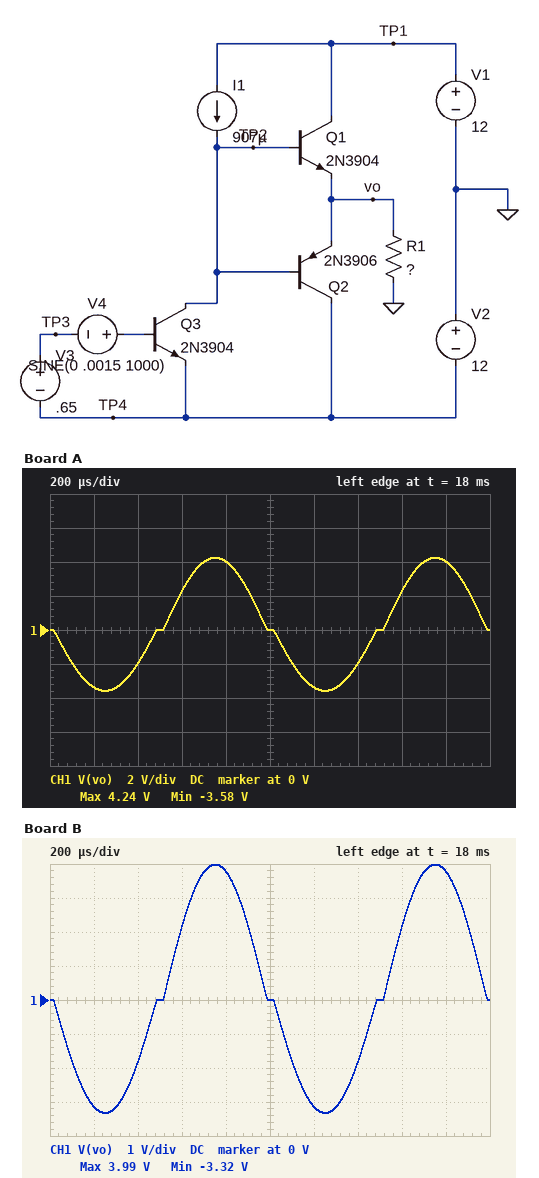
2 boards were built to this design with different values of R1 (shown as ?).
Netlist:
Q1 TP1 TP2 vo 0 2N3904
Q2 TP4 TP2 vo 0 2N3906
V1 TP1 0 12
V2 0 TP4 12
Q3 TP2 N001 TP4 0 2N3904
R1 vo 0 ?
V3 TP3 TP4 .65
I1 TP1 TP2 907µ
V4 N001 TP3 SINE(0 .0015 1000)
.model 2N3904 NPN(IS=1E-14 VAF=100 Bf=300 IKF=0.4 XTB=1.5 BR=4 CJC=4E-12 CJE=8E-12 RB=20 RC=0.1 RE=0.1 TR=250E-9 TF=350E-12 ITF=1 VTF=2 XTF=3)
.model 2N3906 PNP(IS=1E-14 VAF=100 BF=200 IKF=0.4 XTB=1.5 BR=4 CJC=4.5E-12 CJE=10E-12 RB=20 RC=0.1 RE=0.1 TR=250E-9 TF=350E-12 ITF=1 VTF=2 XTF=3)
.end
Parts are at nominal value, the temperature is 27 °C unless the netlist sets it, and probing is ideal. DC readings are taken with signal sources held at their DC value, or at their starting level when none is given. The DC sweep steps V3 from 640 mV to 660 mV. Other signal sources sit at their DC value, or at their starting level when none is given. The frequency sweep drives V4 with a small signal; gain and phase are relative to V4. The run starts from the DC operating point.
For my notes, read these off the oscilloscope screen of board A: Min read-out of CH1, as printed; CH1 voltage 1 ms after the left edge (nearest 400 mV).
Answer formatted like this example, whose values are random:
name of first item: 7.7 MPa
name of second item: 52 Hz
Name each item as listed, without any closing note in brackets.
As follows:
Min read-out of CH1, as printed: -3.58 V
CH1 voltage 1 ms after the left edge: 0 V
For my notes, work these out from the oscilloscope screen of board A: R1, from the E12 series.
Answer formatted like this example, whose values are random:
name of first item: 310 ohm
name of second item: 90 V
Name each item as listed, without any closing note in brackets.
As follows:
R1, from the E12 series: 1 kΩ
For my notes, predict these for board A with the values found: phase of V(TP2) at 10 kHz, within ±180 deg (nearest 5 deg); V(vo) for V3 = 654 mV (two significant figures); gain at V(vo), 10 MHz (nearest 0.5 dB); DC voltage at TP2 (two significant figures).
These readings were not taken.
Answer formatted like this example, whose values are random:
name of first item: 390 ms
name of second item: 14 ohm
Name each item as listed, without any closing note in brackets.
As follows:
phase of V(TP2) at 10 kHz, within ±180 deg: 170 deg
V(vo) for V3 = 654 mV: -9.9 V
gain at V(vo), 10 MHz: 28.0 dB
DC voltage at TP2: 45 mV
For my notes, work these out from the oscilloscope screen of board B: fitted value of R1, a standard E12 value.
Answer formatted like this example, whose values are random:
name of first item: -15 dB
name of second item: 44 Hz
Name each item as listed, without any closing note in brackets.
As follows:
fitted value of R1, a standard E12 value: 820 Ω
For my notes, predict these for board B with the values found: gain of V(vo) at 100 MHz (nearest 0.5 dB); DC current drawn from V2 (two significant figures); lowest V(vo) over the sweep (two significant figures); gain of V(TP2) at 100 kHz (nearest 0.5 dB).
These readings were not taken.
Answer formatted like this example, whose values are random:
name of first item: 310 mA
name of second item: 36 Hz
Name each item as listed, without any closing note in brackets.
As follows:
gain of V(vo) at 100 MHz: 18.0 dB
DC current drawn from V2: 910 µA
lowest V(vo) over the sweep: -11 V
gain of V(TP2) at 100 kHz: 66.0 dB
